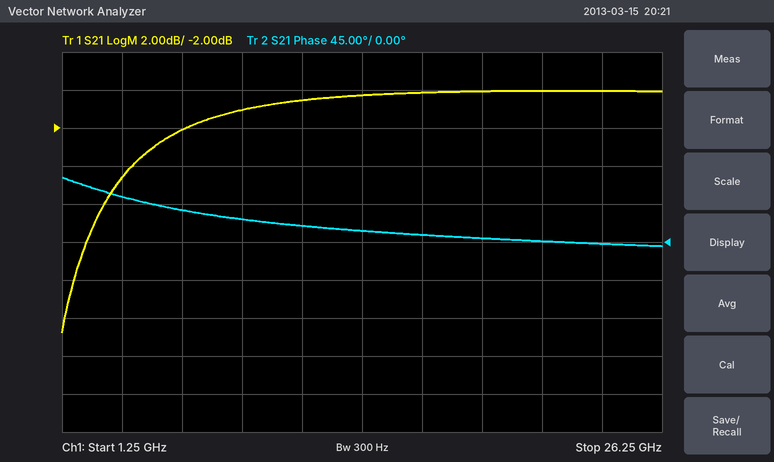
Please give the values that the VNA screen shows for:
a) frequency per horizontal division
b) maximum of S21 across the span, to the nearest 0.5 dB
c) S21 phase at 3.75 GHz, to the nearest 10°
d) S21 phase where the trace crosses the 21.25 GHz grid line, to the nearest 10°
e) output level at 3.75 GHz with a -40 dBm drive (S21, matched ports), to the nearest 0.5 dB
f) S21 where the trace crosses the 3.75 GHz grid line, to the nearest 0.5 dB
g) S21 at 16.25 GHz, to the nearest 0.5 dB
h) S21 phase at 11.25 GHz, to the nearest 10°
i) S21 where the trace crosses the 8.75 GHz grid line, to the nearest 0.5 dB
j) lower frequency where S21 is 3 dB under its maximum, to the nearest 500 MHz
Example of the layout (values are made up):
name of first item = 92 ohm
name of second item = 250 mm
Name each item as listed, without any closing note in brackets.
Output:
frequency per horizontal division = 2.5 GHz
maximum of S21 across the span, to the nearest 0.5 dB = 0.0 dB
S21 phase at 3.75 GHz, to the nearest 10° = 50°
S21 phase where the trace crosses the 21.25 GHz grid line, to the nearest 10° = 0°
output level at 3.75 GHz with a -40 dBm drive (S21, matched ports), to the nearest 0.5 dB = -44.5 dBm
S21 where the trace crosses the 3.75 GHz grid line, to the nearest 0.5 dB = -4.5 dB
S21 at 16.25 GHz, to the nearest 0.5 dB = 0.0 dB
S21 phase at 11.25 GHz, to the nearest 10° = 20°
S21 where the trace crosses the 8.75 GHz grid line, to the nearest 0.5 dB = -1.0 dB
lower frequency where S21 is 3 dB under its maximum, to the nearest 500 MHz = 5.0 GHz
